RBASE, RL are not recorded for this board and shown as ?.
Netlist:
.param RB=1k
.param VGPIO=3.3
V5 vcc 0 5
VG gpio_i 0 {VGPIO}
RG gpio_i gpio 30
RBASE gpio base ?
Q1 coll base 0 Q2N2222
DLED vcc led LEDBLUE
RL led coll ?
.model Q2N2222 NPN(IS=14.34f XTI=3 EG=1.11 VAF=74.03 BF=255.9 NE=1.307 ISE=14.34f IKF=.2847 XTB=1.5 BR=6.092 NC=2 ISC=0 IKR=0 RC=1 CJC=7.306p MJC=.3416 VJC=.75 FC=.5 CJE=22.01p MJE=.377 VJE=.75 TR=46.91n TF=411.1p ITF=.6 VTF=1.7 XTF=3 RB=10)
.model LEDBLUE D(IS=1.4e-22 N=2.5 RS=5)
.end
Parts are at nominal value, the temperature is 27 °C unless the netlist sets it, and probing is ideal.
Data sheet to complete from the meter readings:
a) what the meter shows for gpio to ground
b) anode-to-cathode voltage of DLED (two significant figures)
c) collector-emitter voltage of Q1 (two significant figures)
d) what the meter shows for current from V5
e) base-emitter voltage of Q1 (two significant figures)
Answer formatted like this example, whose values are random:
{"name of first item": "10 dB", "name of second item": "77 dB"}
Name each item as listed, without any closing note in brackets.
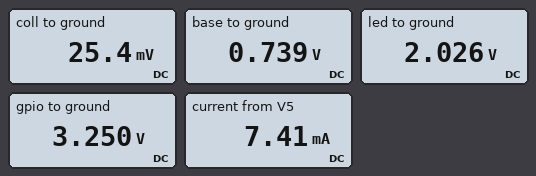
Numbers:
{"what the meter shows for gpio to ground": "3.250 V", "anode-to-cathode voltage of DLED": "3.0 V", "collector-emitter voltage of Q1": "25 mV", "what the meter shows for current from V5": "7.41 mA", "base-emitter voltage of Q1": "740 mV"}
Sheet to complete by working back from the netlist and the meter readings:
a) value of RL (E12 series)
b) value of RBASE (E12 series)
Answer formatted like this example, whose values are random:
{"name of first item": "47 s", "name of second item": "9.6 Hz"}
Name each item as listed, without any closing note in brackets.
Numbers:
{"value of RL": "270 Ω", "value of RBASE": "1.5 kΩ"}
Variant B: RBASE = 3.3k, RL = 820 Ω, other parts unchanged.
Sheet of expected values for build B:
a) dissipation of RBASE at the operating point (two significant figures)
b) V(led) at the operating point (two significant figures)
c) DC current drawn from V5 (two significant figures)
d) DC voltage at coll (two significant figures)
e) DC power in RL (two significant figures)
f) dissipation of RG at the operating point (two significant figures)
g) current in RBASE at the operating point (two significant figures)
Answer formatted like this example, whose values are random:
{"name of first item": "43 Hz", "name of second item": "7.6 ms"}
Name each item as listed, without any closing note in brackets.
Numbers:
{"dissipation of RBASE at the operating point": "2.0 mW", "V(led) at the operating point": "2.1 V", "DC current drawn from V5": "2.6 mA", "DC voltage at coll": "17 mV", "DC power in RL": "5.4 mW", "dissipation of RG at the operating point": "18 µW", "current in RBASE at the operating point": "780 µA"}
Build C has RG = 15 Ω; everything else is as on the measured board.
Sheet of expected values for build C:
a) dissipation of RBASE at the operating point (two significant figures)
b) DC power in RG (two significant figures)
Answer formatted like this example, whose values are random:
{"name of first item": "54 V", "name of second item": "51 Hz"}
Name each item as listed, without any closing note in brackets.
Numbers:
{"dissipation of RBASE at the operating point": "4.3 mW", "DC power in RG": "43 µW"}
